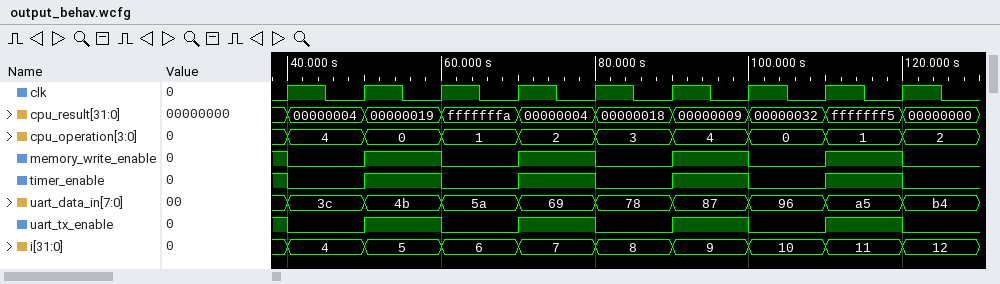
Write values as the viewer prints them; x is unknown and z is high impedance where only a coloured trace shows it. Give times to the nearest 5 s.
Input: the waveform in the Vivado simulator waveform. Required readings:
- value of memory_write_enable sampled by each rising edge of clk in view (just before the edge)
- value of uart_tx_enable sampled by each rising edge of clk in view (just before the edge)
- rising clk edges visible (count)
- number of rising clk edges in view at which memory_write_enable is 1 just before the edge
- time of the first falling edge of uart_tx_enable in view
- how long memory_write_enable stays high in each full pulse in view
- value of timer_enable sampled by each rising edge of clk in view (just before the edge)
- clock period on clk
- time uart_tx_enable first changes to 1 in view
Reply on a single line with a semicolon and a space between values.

1 0 1 0 1 0 1 0 1; 1 0 1 0 1 0 1 0 1; 9; 5; 40 s; 10 s, 10 s, 10 s, 10 s; 1 0 1 0 1 0 1 0 1; 10 s; 50 s
